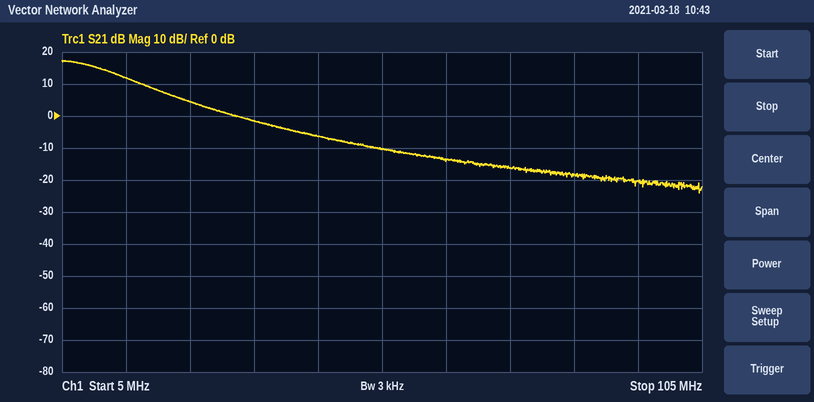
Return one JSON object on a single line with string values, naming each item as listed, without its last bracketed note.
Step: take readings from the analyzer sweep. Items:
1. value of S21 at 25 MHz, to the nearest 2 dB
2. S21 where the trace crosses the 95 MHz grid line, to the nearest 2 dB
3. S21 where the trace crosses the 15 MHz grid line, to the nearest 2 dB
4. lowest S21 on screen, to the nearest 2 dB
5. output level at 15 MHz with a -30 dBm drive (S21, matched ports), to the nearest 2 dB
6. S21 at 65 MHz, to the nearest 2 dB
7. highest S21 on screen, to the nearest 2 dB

{"value of S21 at 25 MHz, to the nearest 2 dB": "4 dB", "S21 where the trace crosses the 95 MHz grid line, to the nearest 2 dB": "-20 dB", "S21 where the trace crosses the 15 MHz grid line, to the nearest 2 dB": "12 dB", "lowest S21 on screen, to the nearest 2 dB": "-24 dB", "output level at 15 MHz with a -30 dBm drive (S21, matched ports), to the nearest 2 dB": "-18 dBm", "S21 at 65 MHz, to the nearest 2 dB": "-14 dB", "highest S21 on screen, to the nearest 2 dB": "18 dB"}
